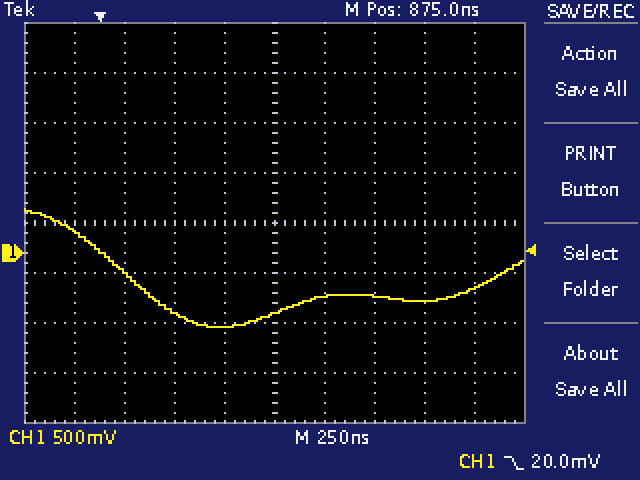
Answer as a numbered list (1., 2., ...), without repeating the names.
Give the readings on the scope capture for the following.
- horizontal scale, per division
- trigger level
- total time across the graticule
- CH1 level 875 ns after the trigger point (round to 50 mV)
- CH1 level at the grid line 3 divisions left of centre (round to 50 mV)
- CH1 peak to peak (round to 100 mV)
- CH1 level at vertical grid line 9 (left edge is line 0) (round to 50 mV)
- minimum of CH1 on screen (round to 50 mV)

1. 250 ns
2. 20.0 mV
3. 2.5 µs
4. -600 mV
5. -200 mV
6. 1.20 V
7. -350 mV
8. -750 mV
